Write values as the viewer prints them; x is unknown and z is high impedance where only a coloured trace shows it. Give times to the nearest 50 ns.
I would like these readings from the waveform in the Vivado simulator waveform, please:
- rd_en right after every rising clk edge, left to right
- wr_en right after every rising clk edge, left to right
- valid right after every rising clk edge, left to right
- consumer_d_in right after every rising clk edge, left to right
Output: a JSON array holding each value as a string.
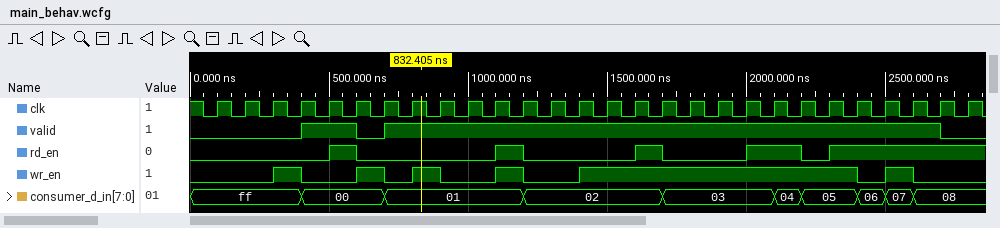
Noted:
["0 0 0 0 1 0 0 0 0 0 1 0 0 0 0 1 0 0 0 1 1 0 1 1 1 1 1 1", "0 0 1 0 0 1 0 1 0 0 1 0 0 1 1 1 1 1 1 1 1 1 1 0 1 0 0 0", "0 0 0 1 1 0 1 1 1 1 1 1 1 1 1 1 1 1 1 1 1 1 1 1 1 1 0 0", "ff, ff, ff, 00, 00, 00, 01, 01, 01, 01, 01, 02, 02, 02, 02, 02, 03, 03, 03, 03, 04, 05, 05, 06, 07, 08, 08, 08"]
